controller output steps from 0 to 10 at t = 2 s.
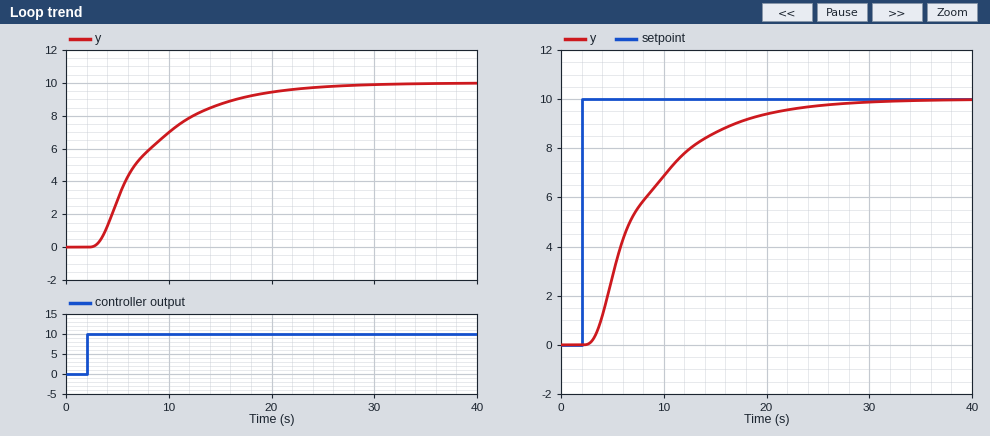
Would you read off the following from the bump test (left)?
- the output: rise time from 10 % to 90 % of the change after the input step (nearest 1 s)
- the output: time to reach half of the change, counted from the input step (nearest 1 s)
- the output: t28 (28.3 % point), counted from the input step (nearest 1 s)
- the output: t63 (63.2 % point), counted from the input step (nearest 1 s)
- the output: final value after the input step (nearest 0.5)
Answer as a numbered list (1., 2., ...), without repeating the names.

1. 13 s
2. 5 s
3. 3 s
4. 7 s
5. 10.0
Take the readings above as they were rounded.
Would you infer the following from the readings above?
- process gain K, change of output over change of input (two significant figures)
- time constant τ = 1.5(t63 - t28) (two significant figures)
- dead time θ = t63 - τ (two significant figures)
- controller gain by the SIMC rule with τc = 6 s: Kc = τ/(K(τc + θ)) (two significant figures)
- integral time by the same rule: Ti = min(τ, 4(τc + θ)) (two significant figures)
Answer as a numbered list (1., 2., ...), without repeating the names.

1. 1.0
2. 6.0 s
3. 1.0 s
4. 0.86
5. 6.0 s
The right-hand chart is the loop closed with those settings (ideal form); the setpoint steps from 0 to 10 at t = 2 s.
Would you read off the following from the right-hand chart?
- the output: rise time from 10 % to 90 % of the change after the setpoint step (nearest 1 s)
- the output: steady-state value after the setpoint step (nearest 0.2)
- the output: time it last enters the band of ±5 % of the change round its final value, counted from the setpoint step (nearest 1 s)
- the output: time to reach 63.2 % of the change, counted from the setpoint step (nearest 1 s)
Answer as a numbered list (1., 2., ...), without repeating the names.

1. 13 s
2. 10.0
3. 19 s
4. 7 s
